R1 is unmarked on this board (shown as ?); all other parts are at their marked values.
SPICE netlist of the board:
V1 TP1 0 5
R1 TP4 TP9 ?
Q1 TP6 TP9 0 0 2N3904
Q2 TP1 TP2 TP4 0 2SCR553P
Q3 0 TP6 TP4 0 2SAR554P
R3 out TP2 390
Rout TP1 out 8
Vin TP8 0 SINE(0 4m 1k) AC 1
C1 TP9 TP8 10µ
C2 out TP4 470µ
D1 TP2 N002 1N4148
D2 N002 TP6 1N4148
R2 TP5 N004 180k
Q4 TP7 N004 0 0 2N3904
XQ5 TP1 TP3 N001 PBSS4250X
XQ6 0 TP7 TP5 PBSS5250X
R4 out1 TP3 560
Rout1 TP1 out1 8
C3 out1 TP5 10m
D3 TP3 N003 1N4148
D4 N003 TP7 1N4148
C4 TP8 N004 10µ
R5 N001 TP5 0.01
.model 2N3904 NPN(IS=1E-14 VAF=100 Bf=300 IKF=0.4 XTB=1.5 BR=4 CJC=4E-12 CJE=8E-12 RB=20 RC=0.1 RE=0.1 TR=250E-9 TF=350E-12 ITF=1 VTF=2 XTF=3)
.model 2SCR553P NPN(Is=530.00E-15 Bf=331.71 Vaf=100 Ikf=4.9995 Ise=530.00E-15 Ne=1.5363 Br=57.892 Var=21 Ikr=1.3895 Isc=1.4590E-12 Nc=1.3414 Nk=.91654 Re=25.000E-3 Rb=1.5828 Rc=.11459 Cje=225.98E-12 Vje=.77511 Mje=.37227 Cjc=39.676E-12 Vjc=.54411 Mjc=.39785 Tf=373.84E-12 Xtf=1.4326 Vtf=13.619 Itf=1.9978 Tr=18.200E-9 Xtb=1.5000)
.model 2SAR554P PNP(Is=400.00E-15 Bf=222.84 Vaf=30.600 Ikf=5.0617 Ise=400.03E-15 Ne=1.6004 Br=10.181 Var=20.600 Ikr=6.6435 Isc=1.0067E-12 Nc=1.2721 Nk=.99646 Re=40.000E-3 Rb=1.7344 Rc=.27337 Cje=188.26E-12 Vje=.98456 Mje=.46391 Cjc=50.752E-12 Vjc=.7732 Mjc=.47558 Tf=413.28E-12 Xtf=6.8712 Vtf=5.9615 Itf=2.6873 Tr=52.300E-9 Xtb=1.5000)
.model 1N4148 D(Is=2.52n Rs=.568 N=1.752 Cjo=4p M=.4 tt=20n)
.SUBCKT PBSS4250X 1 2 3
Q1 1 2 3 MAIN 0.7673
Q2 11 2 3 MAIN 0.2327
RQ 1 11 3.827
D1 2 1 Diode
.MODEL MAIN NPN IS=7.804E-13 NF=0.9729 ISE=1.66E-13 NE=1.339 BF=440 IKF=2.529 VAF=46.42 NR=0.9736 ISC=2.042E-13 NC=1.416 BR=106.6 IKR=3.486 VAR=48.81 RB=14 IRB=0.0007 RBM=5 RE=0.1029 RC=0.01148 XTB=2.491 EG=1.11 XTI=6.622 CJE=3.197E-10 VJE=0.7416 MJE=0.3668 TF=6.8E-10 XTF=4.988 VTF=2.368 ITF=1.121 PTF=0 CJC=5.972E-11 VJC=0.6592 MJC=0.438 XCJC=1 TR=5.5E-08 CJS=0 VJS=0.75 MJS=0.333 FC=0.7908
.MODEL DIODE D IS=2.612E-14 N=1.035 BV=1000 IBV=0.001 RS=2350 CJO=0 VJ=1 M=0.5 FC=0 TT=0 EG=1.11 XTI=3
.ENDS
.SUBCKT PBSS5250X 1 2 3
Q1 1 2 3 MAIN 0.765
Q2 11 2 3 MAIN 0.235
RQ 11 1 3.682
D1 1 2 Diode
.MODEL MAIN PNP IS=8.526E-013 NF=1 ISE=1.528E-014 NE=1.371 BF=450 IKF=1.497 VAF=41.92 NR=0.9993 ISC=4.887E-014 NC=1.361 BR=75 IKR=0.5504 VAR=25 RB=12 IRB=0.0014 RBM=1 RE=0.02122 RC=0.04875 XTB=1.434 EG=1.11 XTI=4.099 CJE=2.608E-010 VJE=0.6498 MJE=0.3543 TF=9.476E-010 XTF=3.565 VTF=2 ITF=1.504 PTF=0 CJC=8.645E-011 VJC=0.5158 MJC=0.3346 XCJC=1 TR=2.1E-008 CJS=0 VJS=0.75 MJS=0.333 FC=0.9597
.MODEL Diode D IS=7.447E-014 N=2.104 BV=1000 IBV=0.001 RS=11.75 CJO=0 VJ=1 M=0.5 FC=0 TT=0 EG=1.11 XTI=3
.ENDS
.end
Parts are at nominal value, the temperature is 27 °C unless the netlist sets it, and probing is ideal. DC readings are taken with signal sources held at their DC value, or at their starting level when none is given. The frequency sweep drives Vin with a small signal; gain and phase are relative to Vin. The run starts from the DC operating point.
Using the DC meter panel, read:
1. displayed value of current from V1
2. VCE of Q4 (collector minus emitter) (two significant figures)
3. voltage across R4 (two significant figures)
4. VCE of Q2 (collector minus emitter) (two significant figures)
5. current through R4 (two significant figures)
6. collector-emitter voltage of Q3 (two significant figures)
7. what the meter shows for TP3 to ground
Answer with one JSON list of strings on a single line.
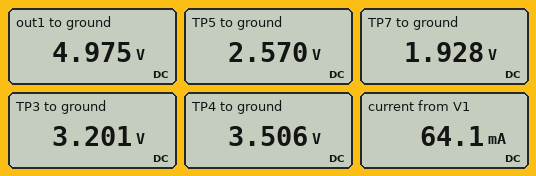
["64.1 mA", "1.9 V", "1.8 V", "1.5 V", "3.2 mA", "-3.5 V", "3.201 V"]
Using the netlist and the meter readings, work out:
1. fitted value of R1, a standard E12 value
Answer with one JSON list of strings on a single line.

["390 kΩ"]
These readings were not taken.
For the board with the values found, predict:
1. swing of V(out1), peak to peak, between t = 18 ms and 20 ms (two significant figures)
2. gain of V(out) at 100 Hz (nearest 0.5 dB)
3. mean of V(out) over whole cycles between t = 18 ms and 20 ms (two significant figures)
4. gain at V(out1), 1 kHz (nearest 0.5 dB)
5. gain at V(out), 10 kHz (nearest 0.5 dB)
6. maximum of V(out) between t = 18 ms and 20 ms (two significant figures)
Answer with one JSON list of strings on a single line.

["2.3 V", "36.0 dB", "5.0 V", "49.5 dB", "40.0 dB", "5.4 V"]
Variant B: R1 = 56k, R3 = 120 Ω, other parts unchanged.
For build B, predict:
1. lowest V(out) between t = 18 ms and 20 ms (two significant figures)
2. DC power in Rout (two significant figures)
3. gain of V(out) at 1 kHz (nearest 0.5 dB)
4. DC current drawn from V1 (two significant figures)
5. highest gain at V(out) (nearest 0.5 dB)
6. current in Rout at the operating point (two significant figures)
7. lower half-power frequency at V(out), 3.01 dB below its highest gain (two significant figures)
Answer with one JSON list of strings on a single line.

["3.2 V", "1.0 mW", "53.0 dB", "230 mA", "54.0 dB", "11 mA", "600 Hz"]
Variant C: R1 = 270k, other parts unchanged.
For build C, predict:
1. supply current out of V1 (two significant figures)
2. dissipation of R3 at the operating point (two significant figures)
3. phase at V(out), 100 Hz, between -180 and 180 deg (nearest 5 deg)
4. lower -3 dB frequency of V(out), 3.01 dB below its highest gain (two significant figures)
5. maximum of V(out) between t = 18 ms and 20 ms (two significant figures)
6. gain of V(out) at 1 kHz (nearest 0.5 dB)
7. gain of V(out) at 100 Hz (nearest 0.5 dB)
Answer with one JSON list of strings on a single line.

["71 mA", "3.2 mW", "-120 deg", "150 Hz", "5.6 V", "43.5 dB", "38.0 dB"]
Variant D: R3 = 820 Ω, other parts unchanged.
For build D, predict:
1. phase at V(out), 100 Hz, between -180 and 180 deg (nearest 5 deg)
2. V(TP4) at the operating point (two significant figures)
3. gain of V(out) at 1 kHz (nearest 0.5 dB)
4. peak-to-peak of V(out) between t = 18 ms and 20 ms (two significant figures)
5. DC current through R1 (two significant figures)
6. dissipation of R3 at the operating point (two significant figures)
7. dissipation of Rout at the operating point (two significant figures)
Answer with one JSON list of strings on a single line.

["-140 deg", "2.9 V", "39.0 dB", "830 mV", "5.8 µA", "2.5 mW", "25 µW"]
